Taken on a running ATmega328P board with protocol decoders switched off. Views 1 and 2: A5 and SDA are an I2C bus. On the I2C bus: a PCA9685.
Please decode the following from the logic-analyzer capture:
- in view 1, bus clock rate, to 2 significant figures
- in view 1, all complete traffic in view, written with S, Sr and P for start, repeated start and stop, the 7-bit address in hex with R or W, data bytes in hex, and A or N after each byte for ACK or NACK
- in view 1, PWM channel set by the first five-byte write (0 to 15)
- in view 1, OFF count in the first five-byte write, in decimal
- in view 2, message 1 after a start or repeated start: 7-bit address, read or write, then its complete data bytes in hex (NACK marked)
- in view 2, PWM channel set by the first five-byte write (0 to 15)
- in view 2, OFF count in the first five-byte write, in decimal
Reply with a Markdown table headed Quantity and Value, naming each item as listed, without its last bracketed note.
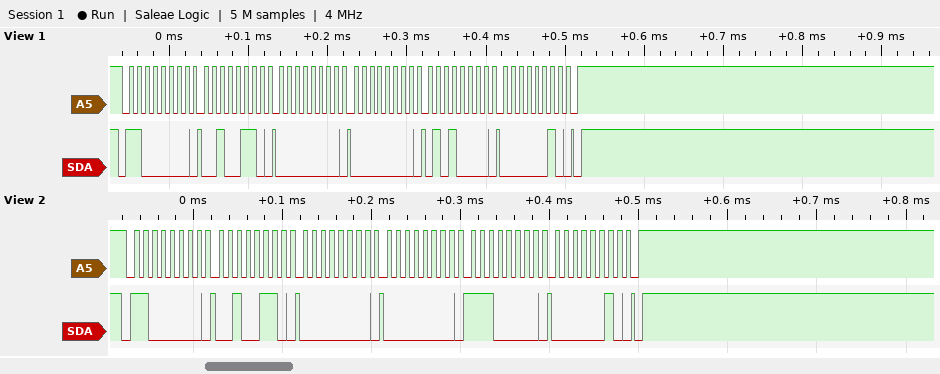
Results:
| Quantity | Value |
|---|---|
| in view 1, bus clock rate, to 2 significant figures | 100 kHz |
| in view 1, all complete traffic in view, written with S, Sr and P for start, repeated start and stop, the 7-bit address in hex with R or W, data bytes in hex, and A or N after each byte for ACK or NACK | S 60W A 26 A 00 A 00 A 50 A 02 A P |
| in view 1, PWM channel set by the first five-byte write | 8 |
| in view 1, OFF count in the first five-byte write, in decimal | 592 |
| in view 2, message 1 after a start or repeated start: 7-bit address, read or write, then its complete data bytes in hex | 0x60 write: 26 00 00 E0 02 |
| in view 2, PWM channel set by the first five-byte write | 8 |
| in view 2, OFF count in the first five-byte write, in decimal | 736 |
